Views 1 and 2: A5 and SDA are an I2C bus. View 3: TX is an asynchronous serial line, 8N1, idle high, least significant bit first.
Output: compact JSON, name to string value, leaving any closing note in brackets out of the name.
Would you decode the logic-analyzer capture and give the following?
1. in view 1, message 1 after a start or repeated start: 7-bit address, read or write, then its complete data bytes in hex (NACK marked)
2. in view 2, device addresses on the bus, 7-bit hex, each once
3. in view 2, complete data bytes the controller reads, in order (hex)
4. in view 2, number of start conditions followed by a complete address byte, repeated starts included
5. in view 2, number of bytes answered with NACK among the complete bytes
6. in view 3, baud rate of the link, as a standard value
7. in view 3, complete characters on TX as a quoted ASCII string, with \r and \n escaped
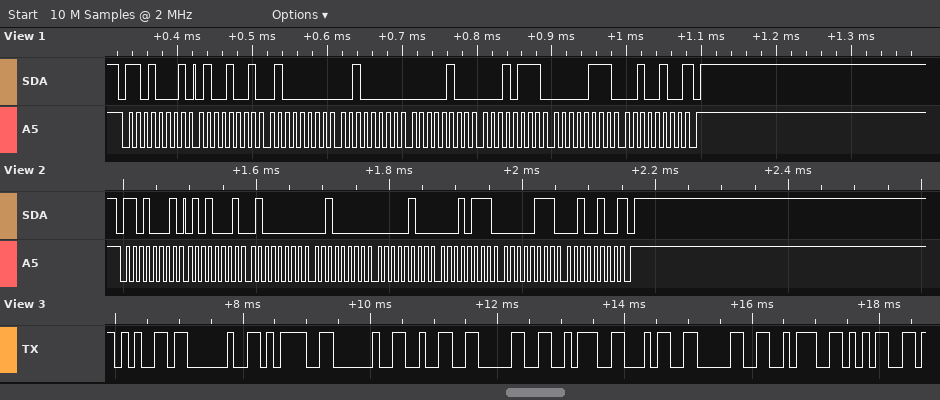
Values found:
{"in view 1, message 1 after a start or repeated start: 7-bit address, read or write, then its complete data bytes in hex": "0x68 read: 49 40 20 04 17 07 24 NACK", "in view 2, device addresses on the bus, 7-bit hex, each once": "0x68", "in view 2, complete data bytes the controller reads, in order": "51 40 20 04 17 07 24", "in view 2, number of start conditions followed by a complete address byte, repeated starts included": "1", "in view 2, number of bytes answered with NACK among the complete bytes": "1", "in view 3, baud rate of the link, as a standard value": "9600 baud", "in view 3, complete characters on TX as a quoted ASCII string, with \\r and \\n escaped": "\"e = 20:40:5\""}
